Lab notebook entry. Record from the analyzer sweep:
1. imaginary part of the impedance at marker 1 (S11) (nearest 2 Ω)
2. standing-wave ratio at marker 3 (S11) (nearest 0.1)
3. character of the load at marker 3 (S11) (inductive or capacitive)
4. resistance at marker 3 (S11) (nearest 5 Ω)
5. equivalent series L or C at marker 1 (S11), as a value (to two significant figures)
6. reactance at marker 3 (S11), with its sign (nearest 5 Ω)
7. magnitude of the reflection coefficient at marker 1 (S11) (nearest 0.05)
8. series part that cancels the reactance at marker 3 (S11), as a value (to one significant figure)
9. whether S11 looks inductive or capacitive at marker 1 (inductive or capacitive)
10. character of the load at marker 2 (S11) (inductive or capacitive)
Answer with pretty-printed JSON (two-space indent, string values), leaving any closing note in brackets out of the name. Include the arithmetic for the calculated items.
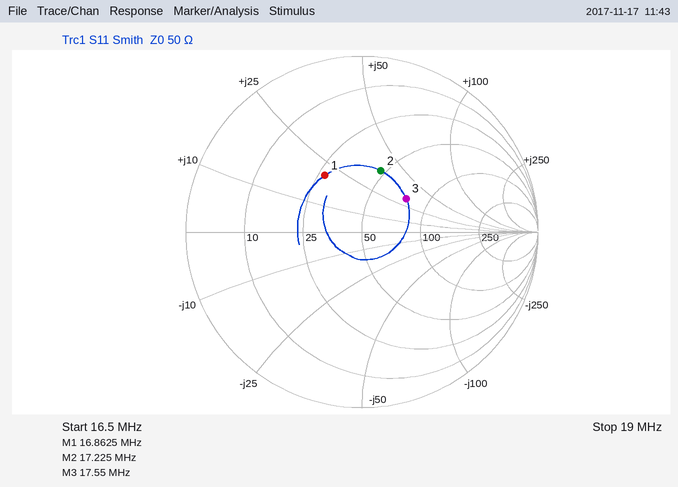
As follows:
{
  "imaginary part of the impedance at marker 1 (S11)": "+20 Ω",
  "standing-wave ratio at marker 3 (S11)": "1.9",
  "character of the load at marker 3 (S11)": "inductive",
  "resistance at marker 3 (S11)": "75 Ω",
  "equivalent series L or C at marker 1 (S11), as a value": "L = 20 Ω/(2π × 16.8625 MHz) ≈ 189 nH, so 190 nH to two significant figures",
  "reactance at marker 3 (S11), with its sign": "+30 Ω",
  "magnitude of the reflection coefficient at marker 1 (S11)": "0.40",
  "series part that cancels the reactance at marker 3 (S11), as a value": "C = 1/(2π × 17.55 MHz × 30 Ω) ≈ 302 pF, so 300 pF to one significant figure",
  "whether S11 looks inductive or capacitive at marker 1": "inductive",
  "character of the load at marker 2 (S11)": "inductive"
}
